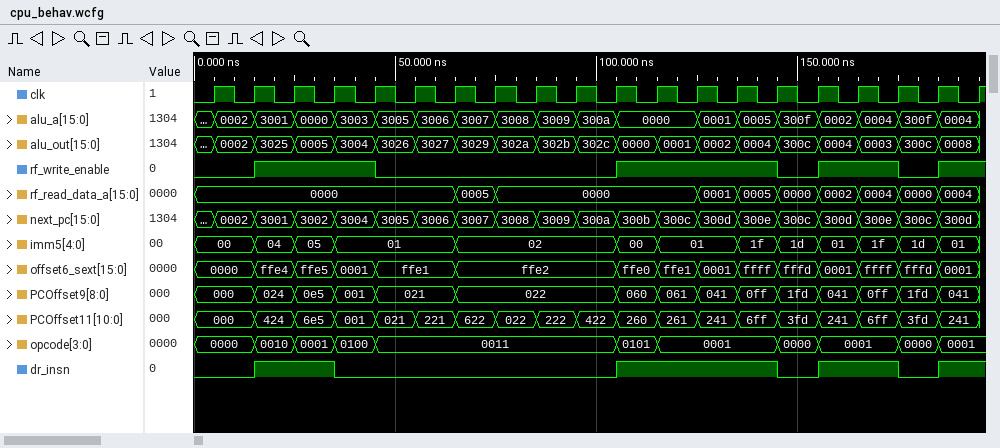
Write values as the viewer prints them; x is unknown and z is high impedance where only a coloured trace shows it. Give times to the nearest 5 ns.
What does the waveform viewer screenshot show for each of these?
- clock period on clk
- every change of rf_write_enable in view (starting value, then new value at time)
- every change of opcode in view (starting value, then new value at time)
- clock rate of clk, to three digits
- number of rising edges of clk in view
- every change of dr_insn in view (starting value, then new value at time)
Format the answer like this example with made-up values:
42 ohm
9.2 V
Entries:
10 ns
0, 1 at 15 ns, 0 at 45 ns, 1 at 105 ns, 0 at 145 ns, 1 at 155 ns, 0 at 175 ns, 1 at 185 ns
0000, 0010 at 15 ns, 0001 at 25 ns, 0100 at 35 ns, 0011 at 45 ns, 0101 at 105 ns, 0001 at 115 ns, 0000 at 145 ns, 0001 at 155 ns, 0000 at 175 ns, 0001 at 185 ns
100 MHz
20
0, 1 at 15 ns, 0 at 35 ns, 1 at 105 ns, 0 at 145 ns, 1 at 155 ns, 0 at 175 ns, 1 at 185 ns
